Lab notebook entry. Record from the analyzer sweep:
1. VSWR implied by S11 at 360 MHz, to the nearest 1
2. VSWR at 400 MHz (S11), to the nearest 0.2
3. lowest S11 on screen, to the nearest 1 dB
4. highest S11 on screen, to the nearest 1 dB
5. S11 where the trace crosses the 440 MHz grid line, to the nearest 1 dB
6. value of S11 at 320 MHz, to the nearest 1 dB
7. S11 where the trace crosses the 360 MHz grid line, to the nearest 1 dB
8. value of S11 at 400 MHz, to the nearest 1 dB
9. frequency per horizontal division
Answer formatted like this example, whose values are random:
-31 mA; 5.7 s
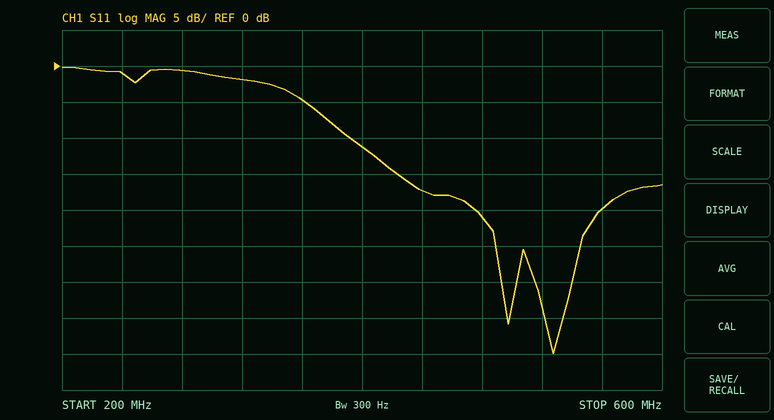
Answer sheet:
4; 1.8; -40 dB; 0 dB; -17 dB; -2 dB; -5 dB; -11 dB; 40 MHz
